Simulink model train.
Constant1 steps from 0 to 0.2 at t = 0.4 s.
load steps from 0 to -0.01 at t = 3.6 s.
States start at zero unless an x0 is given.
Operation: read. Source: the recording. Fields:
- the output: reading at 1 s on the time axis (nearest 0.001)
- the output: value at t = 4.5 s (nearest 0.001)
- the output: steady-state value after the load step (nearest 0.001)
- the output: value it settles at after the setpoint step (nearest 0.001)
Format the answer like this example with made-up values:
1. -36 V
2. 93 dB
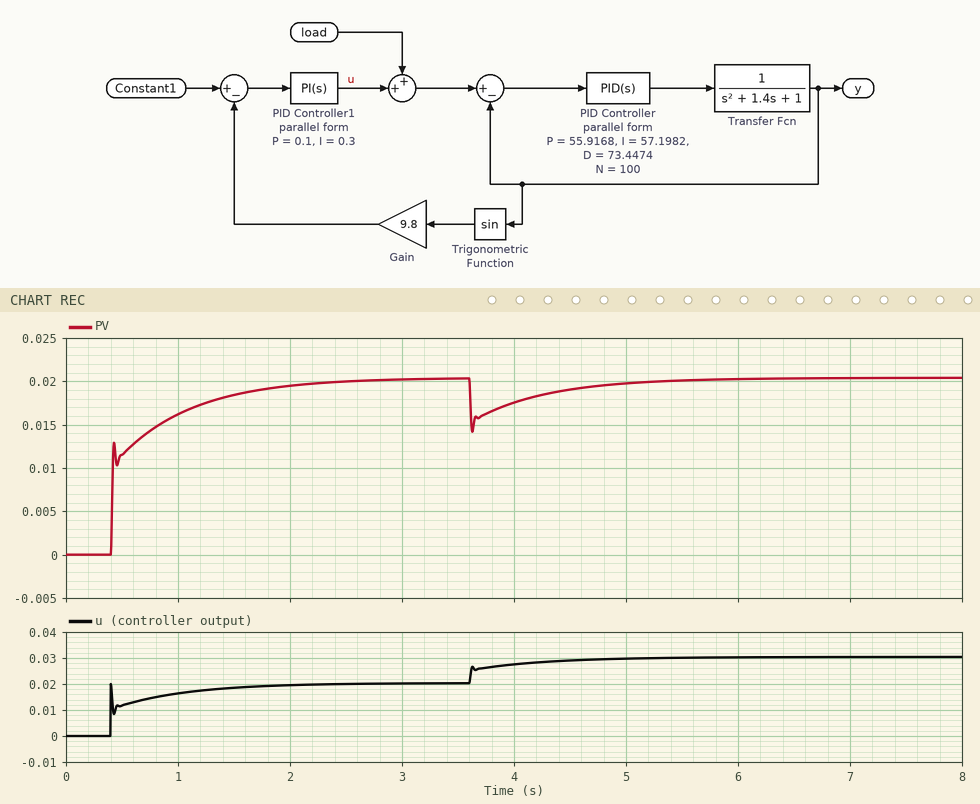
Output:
1. 0.016
2. 0.019
3. 0.020
4. 0.020
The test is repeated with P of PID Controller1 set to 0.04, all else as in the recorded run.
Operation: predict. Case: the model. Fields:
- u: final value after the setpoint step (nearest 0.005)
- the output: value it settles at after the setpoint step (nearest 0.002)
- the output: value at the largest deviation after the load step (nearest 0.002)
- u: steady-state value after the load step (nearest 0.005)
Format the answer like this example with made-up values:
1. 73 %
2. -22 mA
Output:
1. 0.020
2. 0.020
3. 0.012
4. 0.030
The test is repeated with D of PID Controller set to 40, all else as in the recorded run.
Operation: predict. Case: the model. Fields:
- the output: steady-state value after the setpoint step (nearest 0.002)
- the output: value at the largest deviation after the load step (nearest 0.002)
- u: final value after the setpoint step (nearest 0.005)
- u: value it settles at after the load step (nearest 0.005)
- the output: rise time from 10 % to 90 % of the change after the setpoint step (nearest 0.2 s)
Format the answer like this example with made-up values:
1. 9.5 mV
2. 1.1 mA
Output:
1. 0.020
2. 0.014
3. 0.020
4. 0.030
5. 1.0 s
